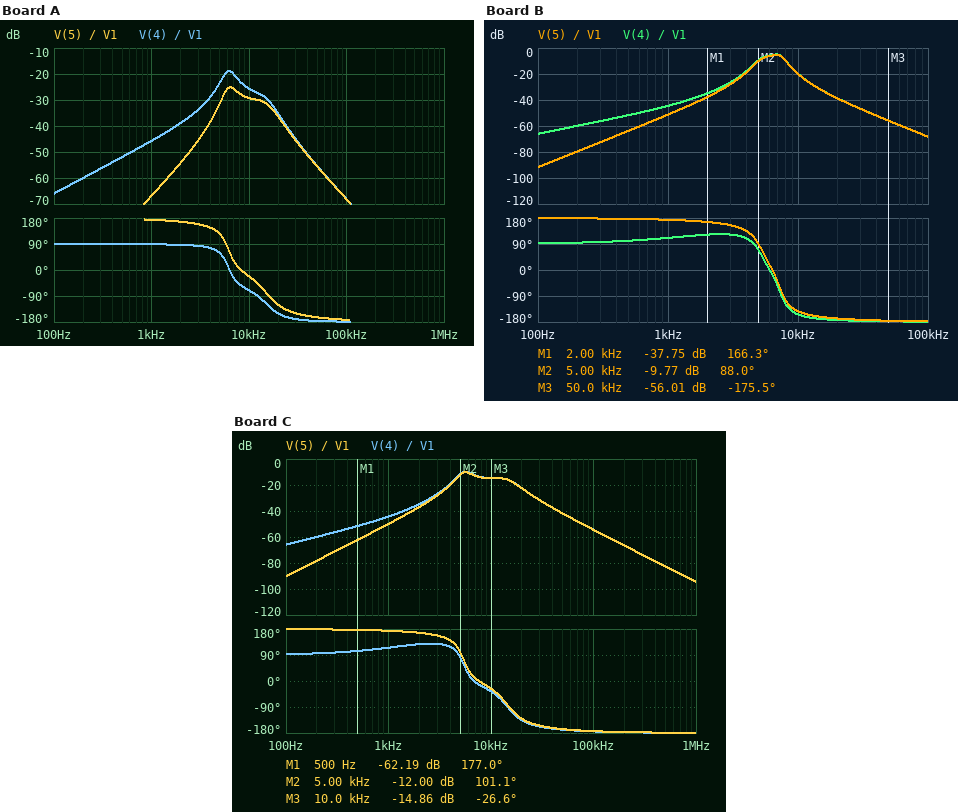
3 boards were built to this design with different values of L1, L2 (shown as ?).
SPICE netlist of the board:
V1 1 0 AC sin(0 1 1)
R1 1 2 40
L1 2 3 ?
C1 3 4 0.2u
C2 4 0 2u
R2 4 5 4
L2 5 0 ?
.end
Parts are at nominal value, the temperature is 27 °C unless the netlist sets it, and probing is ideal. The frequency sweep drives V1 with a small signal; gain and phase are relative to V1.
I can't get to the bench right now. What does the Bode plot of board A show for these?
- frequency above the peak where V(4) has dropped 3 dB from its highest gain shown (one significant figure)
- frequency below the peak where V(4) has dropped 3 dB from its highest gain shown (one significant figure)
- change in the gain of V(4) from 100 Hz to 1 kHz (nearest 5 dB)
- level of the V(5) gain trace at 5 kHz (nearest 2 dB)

8 kHz
5 kHz
20 dB
-32 dB
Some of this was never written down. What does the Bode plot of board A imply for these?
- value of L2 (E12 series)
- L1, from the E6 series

56 µH
3.3 mH
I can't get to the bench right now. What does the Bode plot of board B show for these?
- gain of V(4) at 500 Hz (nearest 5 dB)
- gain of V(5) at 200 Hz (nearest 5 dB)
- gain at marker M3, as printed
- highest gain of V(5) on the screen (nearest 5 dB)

-50 dB
-80 dB
-56.01 dB
-5 dB
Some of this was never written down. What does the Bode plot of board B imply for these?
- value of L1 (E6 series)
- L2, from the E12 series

3.3 mH
330 µH
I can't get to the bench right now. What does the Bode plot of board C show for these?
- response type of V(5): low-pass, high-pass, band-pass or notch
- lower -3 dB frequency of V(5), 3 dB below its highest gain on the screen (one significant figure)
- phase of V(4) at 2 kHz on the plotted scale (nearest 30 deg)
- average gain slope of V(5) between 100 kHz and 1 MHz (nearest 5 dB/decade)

band-pass
5 kHz
120 deg
-40 dB/decade
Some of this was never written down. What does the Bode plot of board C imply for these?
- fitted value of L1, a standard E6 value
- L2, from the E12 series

680 µH
390 µH
